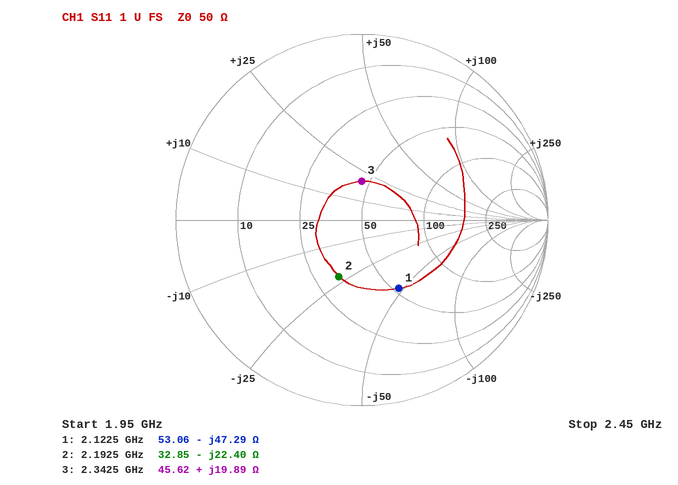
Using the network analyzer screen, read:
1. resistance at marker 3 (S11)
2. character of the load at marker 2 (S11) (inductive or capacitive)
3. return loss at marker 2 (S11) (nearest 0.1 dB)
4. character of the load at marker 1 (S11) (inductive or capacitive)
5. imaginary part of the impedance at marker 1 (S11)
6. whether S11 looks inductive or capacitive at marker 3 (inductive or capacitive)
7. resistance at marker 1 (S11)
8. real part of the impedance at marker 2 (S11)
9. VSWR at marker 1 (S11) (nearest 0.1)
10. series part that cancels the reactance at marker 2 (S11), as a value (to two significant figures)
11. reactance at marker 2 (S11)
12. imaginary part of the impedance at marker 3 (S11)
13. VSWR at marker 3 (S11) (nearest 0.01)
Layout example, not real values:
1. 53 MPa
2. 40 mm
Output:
1. 45.62 Ω
2. capacitive
3. 9.7 dB
4. capacitive
5. -47.29 Ω
6. inductive
7. 53.06 Ω
8. 32.85 Ω
9. 2.4
10. 1.6 nH
11. -22.40 Ω
12. +19.89 Ω
13. 1.53
